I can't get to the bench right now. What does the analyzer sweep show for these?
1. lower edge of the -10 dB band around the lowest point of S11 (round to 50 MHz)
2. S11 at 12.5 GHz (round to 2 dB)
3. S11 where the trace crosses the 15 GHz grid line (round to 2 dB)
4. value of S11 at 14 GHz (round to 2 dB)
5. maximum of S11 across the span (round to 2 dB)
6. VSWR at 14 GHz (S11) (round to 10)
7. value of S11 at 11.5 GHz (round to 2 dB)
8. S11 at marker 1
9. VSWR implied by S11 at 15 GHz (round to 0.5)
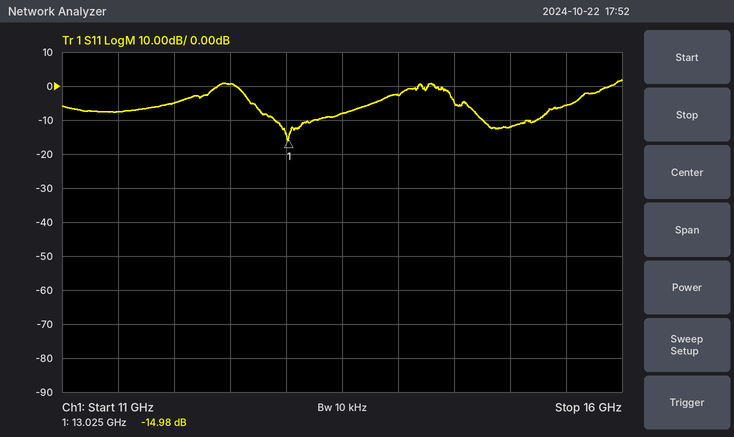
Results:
12.90 GHz
0 dB
-12 dB
-2 dB
2 dB
10
-8 dB
-14.98 dB
1.5
